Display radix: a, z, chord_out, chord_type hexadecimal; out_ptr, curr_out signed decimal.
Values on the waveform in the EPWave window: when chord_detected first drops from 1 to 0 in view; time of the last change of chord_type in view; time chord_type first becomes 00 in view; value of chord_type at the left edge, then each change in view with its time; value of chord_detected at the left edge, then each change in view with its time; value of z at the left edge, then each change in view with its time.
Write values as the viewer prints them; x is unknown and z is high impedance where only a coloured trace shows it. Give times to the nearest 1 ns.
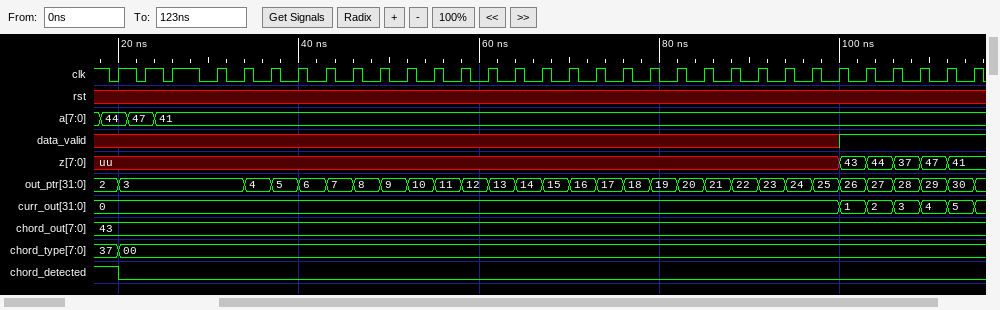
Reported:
20 ns
20 ns
20 ns
37, 00 at 20 ns
1, 0 at 20 ns
uu, 43 at 100 ns, 44 at 103 ns, 37 at 106 ns, 47 at 109 ns, 41 at 112 ns
